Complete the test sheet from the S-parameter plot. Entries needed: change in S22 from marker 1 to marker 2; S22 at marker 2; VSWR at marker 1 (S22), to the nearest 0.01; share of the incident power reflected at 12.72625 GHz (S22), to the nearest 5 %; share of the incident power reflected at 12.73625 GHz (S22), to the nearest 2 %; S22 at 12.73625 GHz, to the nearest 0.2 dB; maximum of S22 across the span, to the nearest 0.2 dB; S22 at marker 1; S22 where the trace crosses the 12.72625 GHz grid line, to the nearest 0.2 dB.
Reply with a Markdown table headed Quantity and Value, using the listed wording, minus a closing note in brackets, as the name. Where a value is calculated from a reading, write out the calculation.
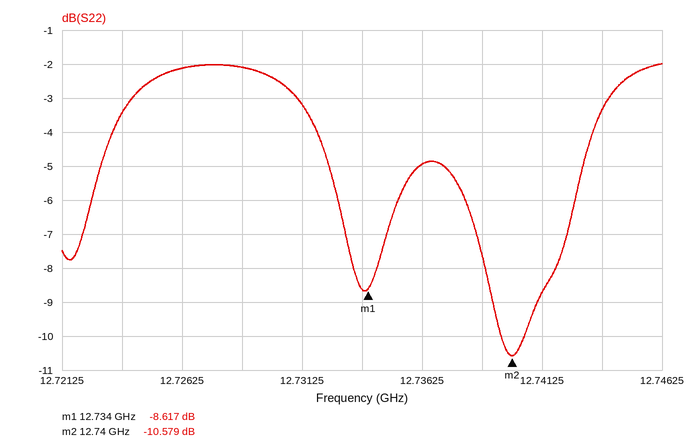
| Quantity | Value |
|---|---|
| change in S22 from marker 1 to marker 2 | -10.579 − (-8.617) = -1.962 dB |
| S22 at marker 2 | -10.579 dB |
| VSWR at marker 1 (S22), to the nearest 0.01 | (1 + 0.3708)/(1 − 0.3708) ≈ 2.18 |
| share of the incident power reflected at 12.72625 GHz (S22), to the nearest 5 % | 10^(-2.2/10) ≈ 60 % |
| share of the incident power reflected at 12.73625 GHz (S22), to the nearest 2 % | 10^(-5/10) ≈ 32 % |
| S22 at 12.73625 GHz, to the nearest 0.2 dB | -5.0 dB |
| maximum of S22 across the span, to the nearest 0.2 dB | -2.0 dB |
| S22 at marker 1 | -8.617 dB |
| S22 where the trace crosses the 12.72625 GHz grid line, to the nearest 0.2 dB | -2.2 dB |
